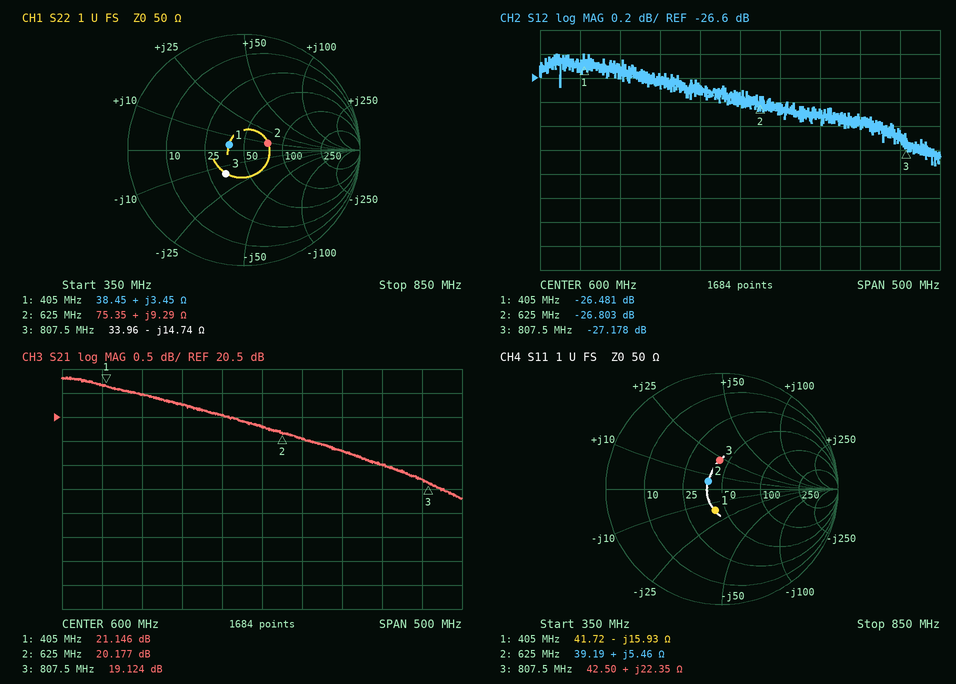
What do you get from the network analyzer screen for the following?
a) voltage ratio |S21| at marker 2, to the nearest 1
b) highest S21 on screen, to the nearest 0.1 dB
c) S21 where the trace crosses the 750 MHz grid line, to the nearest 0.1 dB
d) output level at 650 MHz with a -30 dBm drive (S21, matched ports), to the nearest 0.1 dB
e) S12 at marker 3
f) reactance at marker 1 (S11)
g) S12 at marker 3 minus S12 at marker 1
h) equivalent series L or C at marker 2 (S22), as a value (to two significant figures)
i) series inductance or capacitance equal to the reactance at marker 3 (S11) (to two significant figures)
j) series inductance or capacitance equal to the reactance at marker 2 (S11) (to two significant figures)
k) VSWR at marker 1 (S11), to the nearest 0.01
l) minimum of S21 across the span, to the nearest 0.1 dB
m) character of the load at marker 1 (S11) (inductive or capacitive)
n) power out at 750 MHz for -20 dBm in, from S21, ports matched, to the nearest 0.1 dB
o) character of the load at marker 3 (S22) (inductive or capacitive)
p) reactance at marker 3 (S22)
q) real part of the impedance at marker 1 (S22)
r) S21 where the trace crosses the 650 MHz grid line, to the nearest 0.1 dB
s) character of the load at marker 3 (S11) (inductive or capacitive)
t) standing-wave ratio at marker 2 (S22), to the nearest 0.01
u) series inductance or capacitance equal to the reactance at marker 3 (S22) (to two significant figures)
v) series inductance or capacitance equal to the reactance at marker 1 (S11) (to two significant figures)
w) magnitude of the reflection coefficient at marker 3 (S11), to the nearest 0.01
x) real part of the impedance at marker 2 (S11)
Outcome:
10
21.3 dB
19.5 dB
-10.0 dBm
-27.178 dB
-15.93 Ω
-0.697 dB
2.4 nH
4.4 nH
1.4 nH
1.48
18.8 dB
capacitive
-0.5 dBm
capacitive
-14.74 Ω
38.45 Ω
20.0 dB
inductive
1.55
13 pF
25 pF
0.25
39.19 Ω
